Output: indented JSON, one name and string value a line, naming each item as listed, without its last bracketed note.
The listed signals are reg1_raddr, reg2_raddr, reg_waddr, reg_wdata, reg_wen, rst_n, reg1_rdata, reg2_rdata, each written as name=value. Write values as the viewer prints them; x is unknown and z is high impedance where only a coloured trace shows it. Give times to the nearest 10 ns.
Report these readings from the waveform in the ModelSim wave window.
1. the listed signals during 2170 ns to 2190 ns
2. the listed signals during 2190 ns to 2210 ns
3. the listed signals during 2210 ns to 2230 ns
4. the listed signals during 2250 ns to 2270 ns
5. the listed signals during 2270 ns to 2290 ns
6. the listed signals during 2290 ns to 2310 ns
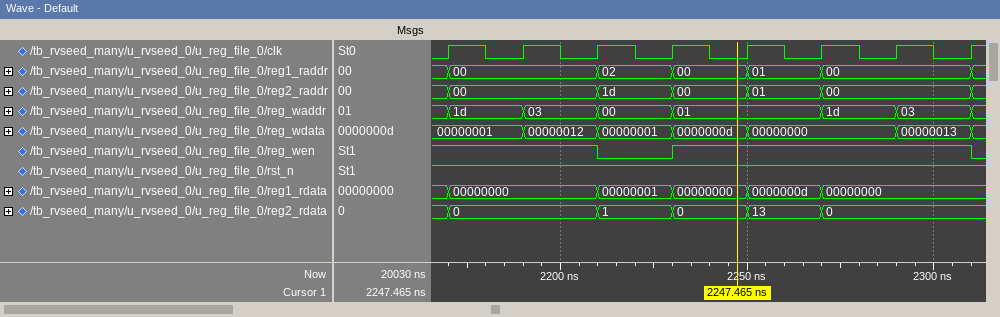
{
  "the listed signals during 2170 ns to 2190 ns": "reg1_raddr=00, reg2_raddr=00, reg_waddr=1d, reg_wdata=00000001, reg_wen=1, rst_n=1, reg1_rdata=00000000, reg2_rdata=0",
  "the listed signals during 2190 ns to 2210 ns": "reg1_raddr=00, reg2_raddr=00, reg_waddr=03, reg_wdata=00000012, reg_wen=1, rst_n=1, reg1_rdata=00000000, reg2_rdata=0",
  "the listed signals during 2210 ns to 2230 ns": "reg1_raddr=02, reg2_raddr=1d, reg_waddr=00, reg_wdata=00000001, reg_wen=0, rst_n=1, reg1_rdata=00000001, reg2_rdata=1",
  "the listed signals during 2250 ns to 2270 ns": "reg1_raddr=01, reg2_raddr=01, reg_waddr=01, reg_wdata=00000000, reg_wen=1, rst_n=1, reg1_rdata=0000000d, reg2_rdata=13",
  "the listed signals during 2270 ns to 2290 ns": "reg1_raddr=00, reg2_raddr=00, reg_waddr=1d, reg_wdata=00000000, reg_wen=1, rst_n=1, reg1_rdata=00000000, reg2_rdata=0",
  "the listed signals during 2290 ns to 2310 ns": "reg1_raddr=00, reg2_raddr=00, reg_waddr=03, reg_wdata=00000013, reg_wen=1, rst_n=1, reg1_rdata=00000000, reg2_rdata=0"
}
